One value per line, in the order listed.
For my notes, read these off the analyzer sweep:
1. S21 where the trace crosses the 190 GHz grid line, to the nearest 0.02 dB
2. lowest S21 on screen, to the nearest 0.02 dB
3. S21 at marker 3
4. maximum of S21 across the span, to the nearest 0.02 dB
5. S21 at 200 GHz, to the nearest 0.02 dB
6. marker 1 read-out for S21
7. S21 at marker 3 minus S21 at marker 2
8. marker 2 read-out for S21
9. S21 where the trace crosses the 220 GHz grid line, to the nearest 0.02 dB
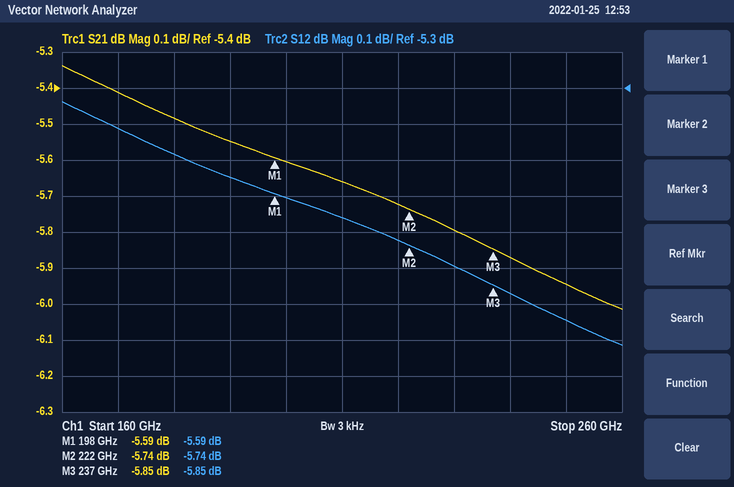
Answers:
-5.54 dB
-6.02 dB
-5.85 dB
-5.34 dB
-5.60 dB
-5.59 dB
-0.11 dB
-5.74 dB
-5.72 dB
